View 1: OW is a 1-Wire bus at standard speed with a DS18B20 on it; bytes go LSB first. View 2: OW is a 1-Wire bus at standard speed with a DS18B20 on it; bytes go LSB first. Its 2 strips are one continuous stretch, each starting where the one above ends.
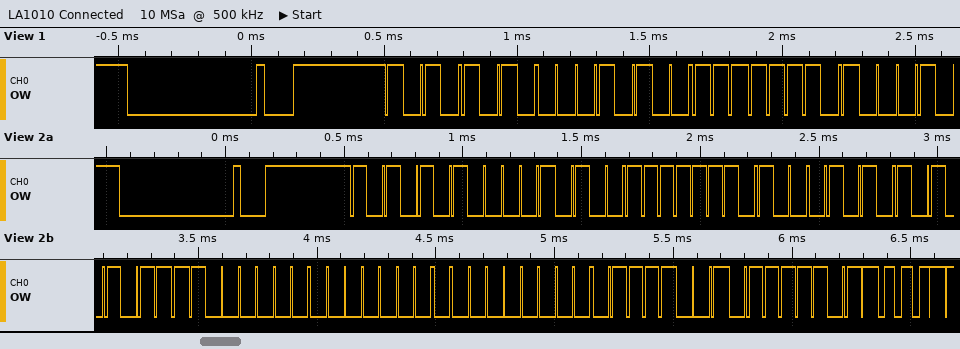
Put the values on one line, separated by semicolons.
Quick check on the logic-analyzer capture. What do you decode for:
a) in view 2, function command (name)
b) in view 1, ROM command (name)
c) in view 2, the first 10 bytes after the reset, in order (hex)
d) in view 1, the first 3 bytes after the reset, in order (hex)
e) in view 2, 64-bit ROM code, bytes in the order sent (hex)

Read Scratchpad; Match ROM; 55 28 7F 51 D5 03 00 00 9E BE; 55 28 7F; 28 7F 51 D5 03 00 00 9E
